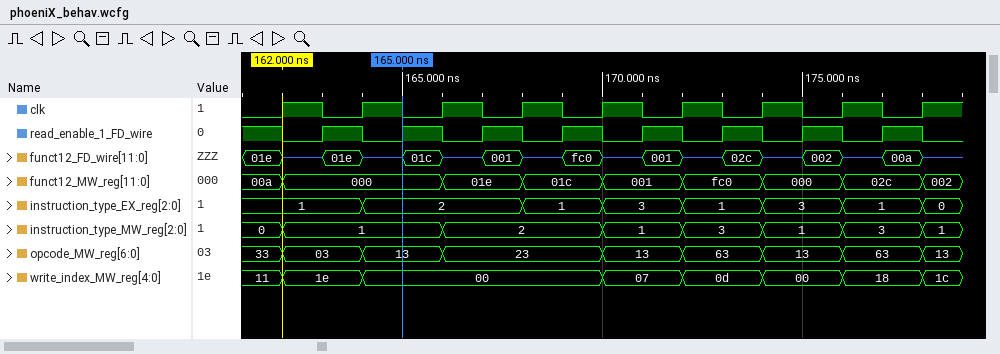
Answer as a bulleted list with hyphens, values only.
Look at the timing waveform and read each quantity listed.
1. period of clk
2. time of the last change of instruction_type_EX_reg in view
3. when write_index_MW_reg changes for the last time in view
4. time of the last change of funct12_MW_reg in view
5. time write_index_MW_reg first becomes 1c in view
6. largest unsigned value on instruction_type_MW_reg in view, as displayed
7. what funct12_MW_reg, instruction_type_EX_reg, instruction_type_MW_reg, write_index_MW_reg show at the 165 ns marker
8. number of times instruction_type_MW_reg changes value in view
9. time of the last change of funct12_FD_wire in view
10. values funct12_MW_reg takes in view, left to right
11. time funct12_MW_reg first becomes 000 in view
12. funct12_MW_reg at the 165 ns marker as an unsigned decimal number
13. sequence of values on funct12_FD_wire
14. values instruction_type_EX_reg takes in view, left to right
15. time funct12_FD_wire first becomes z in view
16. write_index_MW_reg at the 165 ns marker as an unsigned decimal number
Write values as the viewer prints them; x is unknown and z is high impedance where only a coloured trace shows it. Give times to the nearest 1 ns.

- 2 ns
- 178 ns
- 178 ns
- 178 ns
- 178 ns
- 3
- funct12_MW_reg=000, instruction_type_EX_reg=2, instruction_type_MW_reg=1, write_index_MW_reg=00
- 7
- 178 ns
- 00a, 000, 01e, 01c, 001, fc0, 000, 02c, 002
- 162 ns
- 0
- 01e, z, 01e, z, 01c, z, 001, z, fc0, z, 001, z, 02c, z, 002, z, 00a, z
- 1, 2, 1, 3, 1, 3, 1, 0
- 162 ns
- 0
